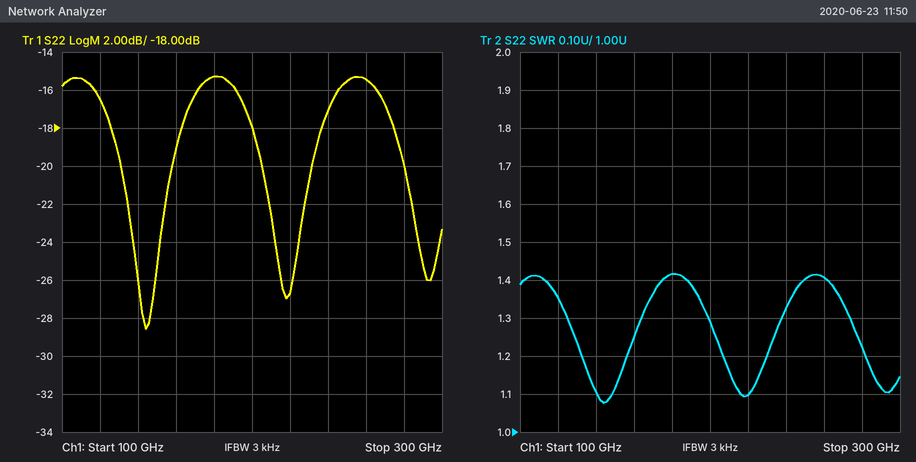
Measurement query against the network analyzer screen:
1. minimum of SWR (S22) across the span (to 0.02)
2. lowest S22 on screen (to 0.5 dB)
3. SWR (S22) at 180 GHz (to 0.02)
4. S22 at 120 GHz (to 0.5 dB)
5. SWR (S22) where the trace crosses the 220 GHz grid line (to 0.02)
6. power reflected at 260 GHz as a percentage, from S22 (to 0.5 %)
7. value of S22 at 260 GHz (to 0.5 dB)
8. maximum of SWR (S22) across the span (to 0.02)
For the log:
1.08
-28.5 dB
1.42
-16.5 dB
1.10
3.0 %
-15.5 dB
1.42
